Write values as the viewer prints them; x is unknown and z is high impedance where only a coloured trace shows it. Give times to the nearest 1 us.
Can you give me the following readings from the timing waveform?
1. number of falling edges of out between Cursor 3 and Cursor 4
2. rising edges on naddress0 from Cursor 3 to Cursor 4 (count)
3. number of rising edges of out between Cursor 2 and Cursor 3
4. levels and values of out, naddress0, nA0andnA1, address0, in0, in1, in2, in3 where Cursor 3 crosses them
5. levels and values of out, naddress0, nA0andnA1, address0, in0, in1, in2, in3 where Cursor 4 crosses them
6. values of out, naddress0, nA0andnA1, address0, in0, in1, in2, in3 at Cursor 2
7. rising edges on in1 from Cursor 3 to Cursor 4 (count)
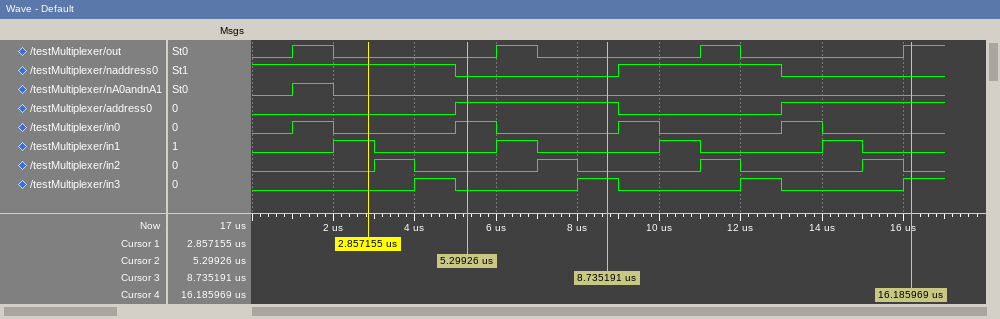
1
1
1
out=0, naddress0=0, nA0andnA1=0, address0=1, in0=0, in1=0, in2=0, in3=1
out=1, naddress0=0, nA0andnA1=0, address0=1, in0=0, in1=0, in2=0, in3=1
out=0, naddress0=0, nA0andnA1=0, address0=1, in0=1, in1=0, in2=0, in3=0
2
